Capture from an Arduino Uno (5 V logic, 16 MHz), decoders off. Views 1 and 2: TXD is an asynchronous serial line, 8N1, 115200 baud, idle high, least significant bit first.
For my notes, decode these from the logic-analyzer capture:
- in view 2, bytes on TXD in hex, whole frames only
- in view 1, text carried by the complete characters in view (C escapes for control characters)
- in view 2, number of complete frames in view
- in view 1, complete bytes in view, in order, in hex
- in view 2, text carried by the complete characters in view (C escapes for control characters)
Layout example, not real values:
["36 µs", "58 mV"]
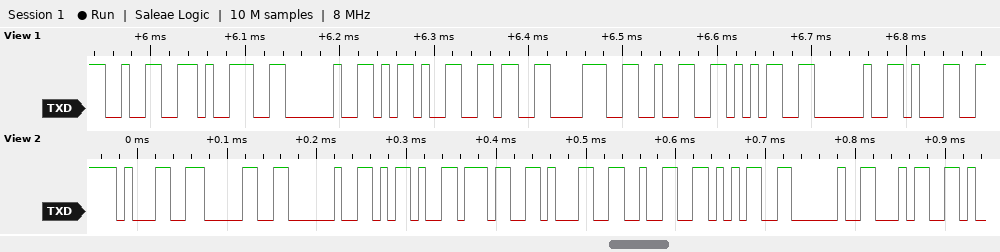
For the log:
["0x31 0x30 0x20 0x2D 0x37 0x31 0x32 0x35 0x20 0x34", "\"29 -6825 1\"", "10", "32 39 20 2D 36 38 32 35 20 31", "\"10 -7125 4\""]
